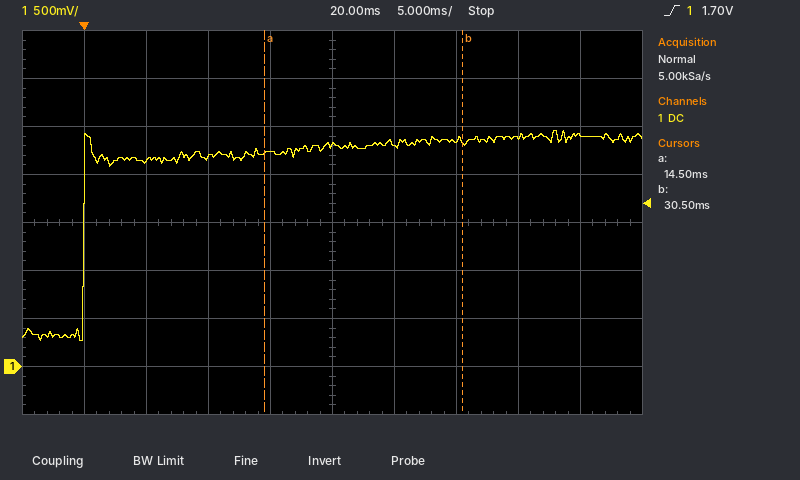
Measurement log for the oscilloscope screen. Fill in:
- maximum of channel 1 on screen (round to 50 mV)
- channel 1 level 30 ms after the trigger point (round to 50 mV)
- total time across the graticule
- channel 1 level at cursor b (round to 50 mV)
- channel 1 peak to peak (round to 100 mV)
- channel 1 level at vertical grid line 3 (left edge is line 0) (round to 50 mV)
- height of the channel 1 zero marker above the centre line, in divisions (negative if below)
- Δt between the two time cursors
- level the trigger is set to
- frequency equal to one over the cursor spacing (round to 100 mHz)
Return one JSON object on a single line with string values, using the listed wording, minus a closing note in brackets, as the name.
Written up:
{"maximum of channel 1 on screen": "2.45 V", "channel 1 level 30 ms after the trigger point": "2.35 V", "total time across the graticule": "50 ms", "channel 1 level at cursor b": "2.35 V", "channel 1 peak to peak": "2.20 V", "channel 1 level at vertical grid line 3 (left edge is line 0)": "2.20 V", "height of the channel 1 zero marker above the centre line, in divisions": "-3.0 div", "Δt between the two time cursors": "16.0 ms", "level the trigger is set to": "1.70 V", "frequency equal to one over the cursor spacing": "62.5 Hz"}
